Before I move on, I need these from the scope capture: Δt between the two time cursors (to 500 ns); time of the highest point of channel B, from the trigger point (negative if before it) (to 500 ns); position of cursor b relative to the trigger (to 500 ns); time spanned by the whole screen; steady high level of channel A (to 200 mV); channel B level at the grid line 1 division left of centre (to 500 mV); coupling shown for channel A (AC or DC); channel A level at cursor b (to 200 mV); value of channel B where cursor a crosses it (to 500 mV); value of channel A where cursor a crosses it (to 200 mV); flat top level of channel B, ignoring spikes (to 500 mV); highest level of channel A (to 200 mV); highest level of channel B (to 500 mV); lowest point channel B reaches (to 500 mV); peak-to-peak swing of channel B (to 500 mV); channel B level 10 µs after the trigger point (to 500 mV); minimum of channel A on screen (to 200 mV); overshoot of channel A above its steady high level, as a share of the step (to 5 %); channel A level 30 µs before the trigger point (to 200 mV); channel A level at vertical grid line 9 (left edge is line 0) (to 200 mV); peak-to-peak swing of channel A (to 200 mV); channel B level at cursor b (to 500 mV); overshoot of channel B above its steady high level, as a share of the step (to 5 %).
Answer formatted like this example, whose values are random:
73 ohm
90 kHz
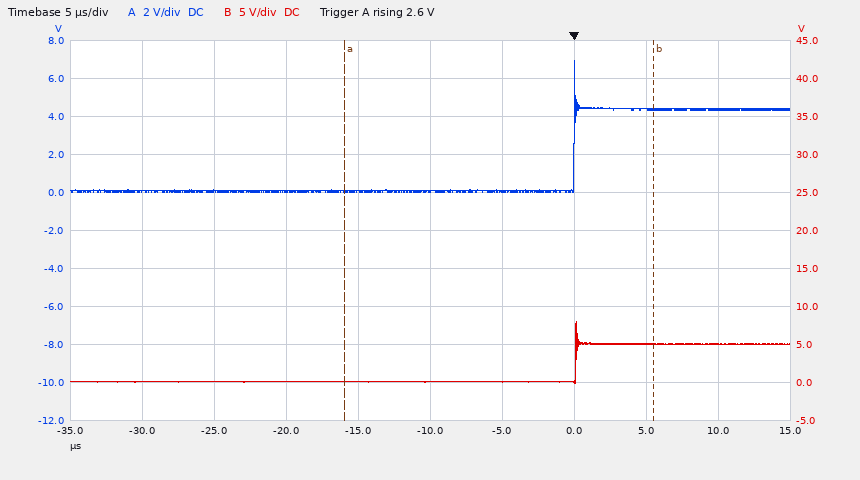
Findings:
21.5 µs
0.0 µs
+5.5 µs
50 µs
4.4 V
0.0 V
DC
4.4 V
0.0 V
0.0 V
5.0 V
7.0 V
8.0 V
0.0 V
8.0 V
5.0 V
0.0 V
60 %
0.0 V
4.4 V
7.0 V
5.0 V
60 %
